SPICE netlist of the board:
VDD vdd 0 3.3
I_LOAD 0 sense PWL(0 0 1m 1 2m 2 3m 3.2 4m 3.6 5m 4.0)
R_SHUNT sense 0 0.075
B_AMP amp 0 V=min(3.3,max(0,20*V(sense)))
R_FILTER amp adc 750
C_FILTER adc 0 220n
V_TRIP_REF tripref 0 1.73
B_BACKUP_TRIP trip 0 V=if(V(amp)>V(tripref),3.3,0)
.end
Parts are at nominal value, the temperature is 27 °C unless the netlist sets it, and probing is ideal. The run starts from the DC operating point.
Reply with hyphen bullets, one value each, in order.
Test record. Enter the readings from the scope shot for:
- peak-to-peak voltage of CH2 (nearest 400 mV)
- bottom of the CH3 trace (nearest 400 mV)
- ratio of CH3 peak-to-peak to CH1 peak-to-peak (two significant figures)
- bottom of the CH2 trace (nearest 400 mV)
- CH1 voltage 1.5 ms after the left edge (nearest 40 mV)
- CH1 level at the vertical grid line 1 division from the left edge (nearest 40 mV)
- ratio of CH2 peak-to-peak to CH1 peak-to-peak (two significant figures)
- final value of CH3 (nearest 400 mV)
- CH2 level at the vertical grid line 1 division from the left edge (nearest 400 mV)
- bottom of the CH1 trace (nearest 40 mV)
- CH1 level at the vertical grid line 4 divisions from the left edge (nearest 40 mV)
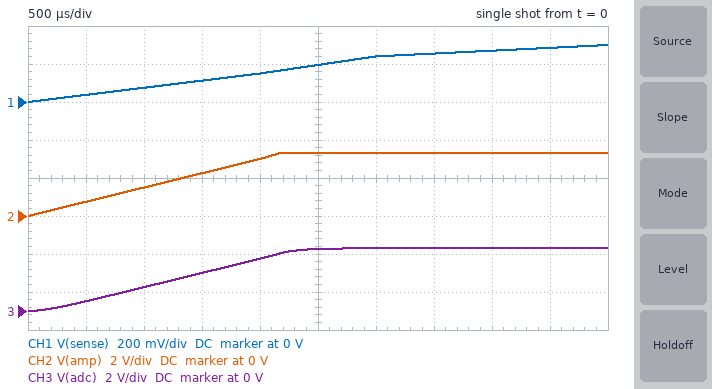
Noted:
- 3.2 V
- 0 V
- 11
- 0 V
- 120 mV
- 40 mV
- 11
- 3.2 V
- 800 mV
- 0 V
- 160 mV
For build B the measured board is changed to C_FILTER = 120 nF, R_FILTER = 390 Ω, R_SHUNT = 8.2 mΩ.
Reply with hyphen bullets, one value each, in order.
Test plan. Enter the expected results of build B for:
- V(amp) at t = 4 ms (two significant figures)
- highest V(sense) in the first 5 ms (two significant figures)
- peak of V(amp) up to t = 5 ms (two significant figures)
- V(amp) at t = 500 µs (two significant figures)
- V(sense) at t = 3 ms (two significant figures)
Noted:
- 590 mV
- 33 mV
- 660 mV
- 82 mV
- 26 mV
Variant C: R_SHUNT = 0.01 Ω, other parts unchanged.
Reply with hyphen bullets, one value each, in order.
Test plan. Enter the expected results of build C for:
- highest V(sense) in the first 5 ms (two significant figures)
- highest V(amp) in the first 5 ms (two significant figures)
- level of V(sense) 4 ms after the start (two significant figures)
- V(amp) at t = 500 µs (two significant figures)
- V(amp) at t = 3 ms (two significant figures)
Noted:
- 40 mV
- 800 mV
- 36 mV
- 100 mV
- 640 mV
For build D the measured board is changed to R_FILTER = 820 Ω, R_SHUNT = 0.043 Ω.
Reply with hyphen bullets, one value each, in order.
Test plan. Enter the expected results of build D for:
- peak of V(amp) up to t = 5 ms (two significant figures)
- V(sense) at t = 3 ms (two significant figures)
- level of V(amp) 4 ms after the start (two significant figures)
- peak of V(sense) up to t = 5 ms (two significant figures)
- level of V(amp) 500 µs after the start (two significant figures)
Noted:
- 3.3 V
- 140 mV
- 3.1 V
- 170 mV
- 430 mV
